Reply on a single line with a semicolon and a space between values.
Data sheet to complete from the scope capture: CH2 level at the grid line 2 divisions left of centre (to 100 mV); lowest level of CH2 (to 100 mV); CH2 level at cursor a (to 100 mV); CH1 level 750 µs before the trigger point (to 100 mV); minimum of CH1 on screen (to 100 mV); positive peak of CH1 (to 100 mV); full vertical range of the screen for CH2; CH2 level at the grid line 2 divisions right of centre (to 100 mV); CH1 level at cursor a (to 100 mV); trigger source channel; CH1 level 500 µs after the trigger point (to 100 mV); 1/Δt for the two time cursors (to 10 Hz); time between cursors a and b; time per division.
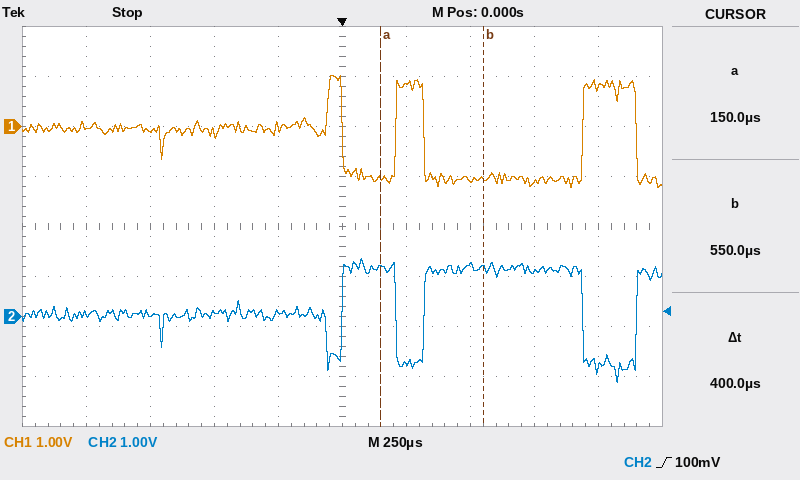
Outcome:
100 mV; -1.3 V; 1.0 V; -100 mV; -1.2 V; 1.0 V; 8 V; 1.0 V; -1.0 V; CH2; -1.1 V; 2.50 kHz; 400 µs; 250 µs
